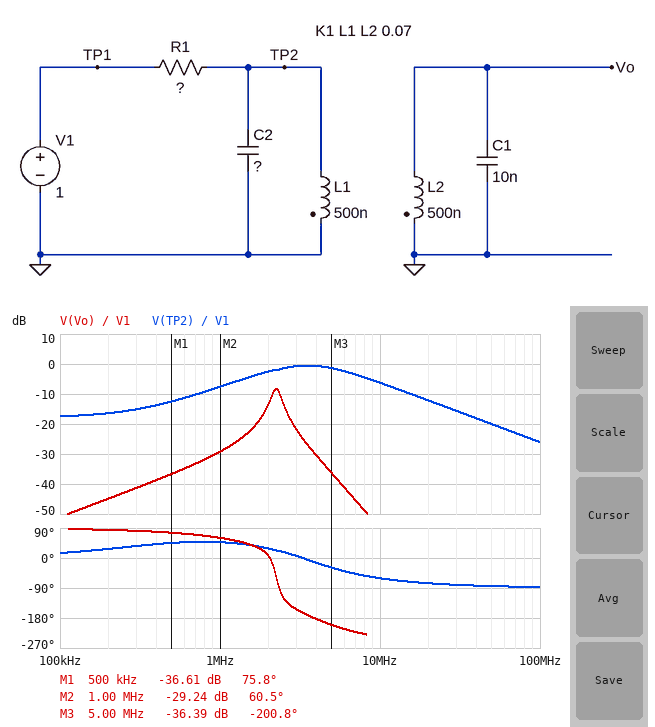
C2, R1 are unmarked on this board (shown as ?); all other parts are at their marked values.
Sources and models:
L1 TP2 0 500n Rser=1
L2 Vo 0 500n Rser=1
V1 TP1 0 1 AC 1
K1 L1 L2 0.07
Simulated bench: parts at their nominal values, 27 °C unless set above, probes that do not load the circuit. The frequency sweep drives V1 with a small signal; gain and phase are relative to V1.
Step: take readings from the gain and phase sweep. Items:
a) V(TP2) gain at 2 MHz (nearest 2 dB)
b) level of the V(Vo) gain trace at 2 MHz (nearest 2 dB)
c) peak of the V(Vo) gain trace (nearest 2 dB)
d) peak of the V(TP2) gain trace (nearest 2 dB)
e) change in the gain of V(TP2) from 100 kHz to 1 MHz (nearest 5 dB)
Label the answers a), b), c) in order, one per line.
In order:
a) -2 dB
b) -14 dB
c) -8 dB
d) 0 dB
e) 10 dB
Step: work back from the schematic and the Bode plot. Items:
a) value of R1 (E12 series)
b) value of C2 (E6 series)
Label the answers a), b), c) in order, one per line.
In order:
a) 6.8 Ω
b) 4.7 nF
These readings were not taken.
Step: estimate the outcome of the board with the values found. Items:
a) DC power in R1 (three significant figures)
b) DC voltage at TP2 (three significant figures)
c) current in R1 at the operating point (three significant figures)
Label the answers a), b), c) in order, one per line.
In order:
a) 112 mW
b) 128 mV
c) 128 mA
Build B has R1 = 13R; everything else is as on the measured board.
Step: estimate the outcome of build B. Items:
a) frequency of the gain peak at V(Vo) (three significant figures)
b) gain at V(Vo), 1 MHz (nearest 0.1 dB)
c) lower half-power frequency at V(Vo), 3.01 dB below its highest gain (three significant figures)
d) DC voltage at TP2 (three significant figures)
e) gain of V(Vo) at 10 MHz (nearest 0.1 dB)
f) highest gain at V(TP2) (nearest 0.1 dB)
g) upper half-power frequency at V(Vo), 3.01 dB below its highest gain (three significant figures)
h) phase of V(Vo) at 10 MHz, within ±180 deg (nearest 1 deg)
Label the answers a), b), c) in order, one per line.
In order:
a) 2.25 MHz
b) -33.7 dB
c) 2.10 MHz
d) 71.4 mV
e) -59.6 dB
f) -1.0 dB
g) 2.43 MHz
h) 110 deg
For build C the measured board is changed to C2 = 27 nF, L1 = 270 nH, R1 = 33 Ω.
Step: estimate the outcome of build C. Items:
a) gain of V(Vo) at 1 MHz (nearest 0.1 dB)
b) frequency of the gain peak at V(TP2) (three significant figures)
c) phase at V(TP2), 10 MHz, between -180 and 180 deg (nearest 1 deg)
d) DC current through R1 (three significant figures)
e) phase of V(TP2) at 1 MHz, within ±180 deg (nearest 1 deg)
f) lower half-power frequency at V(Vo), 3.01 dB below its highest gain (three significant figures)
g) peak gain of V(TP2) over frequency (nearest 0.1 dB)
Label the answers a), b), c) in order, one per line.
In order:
a) -42.1 dB
b) 1.87 MHz
c) -89 deg
d) 29.4 mA
e) 43 deg
f) 1.98 MHz
g) -12.3 dB
